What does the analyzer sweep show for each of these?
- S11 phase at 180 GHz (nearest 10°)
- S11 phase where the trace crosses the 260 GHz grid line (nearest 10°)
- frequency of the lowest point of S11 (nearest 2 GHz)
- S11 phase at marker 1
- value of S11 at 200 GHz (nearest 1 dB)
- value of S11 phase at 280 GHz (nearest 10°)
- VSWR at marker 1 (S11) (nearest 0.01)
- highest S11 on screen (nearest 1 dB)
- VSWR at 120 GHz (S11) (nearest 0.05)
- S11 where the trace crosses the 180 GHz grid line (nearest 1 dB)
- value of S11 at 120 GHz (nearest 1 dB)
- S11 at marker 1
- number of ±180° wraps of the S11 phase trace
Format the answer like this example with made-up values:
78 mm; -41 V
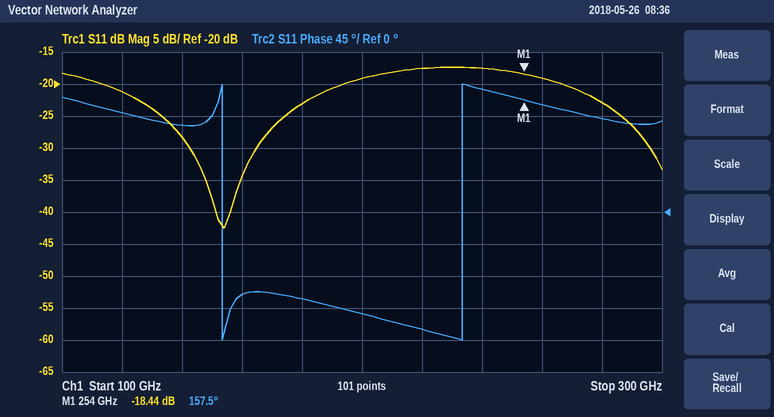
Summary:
-120°; 150°; 154 GHz; 157.5°; -19 dB; 130°; 1.27; -17 dB; 1.20; -23 dB; -21 dB; -18.44 dB; 2
